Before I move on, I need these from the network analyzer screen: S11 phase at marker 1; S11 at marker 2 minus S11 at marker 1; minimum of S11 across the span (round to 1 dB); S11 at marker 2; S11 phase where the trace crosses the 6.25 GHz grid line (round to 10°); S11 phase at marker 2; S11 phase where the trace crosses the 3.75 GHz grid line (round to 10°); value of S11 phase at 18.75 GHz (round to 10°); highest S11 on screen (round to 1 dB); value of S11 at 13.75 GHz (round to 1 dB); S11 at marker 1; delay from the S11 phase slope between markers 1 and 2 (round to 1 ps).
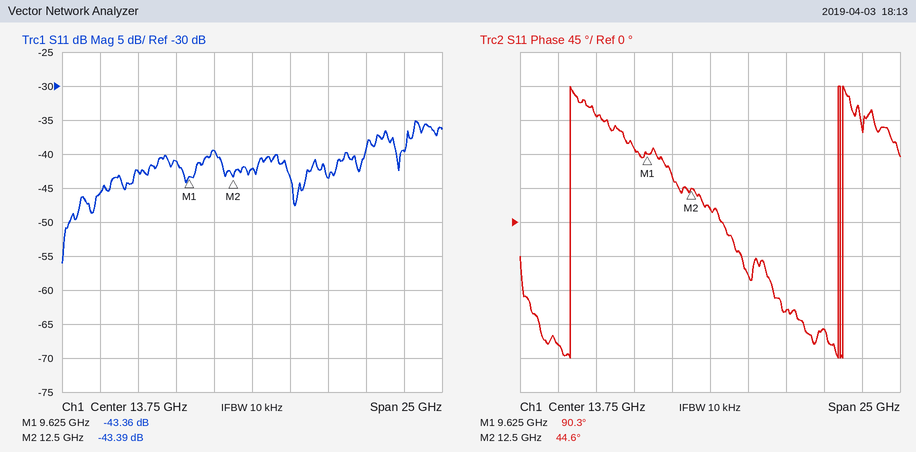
90.3°
-0.03 dB
-56 dB
-43.39 dB
140°
44.6°
-160°
-120°
-35 dB
-42 dB
-43.36 dB
44 ps
